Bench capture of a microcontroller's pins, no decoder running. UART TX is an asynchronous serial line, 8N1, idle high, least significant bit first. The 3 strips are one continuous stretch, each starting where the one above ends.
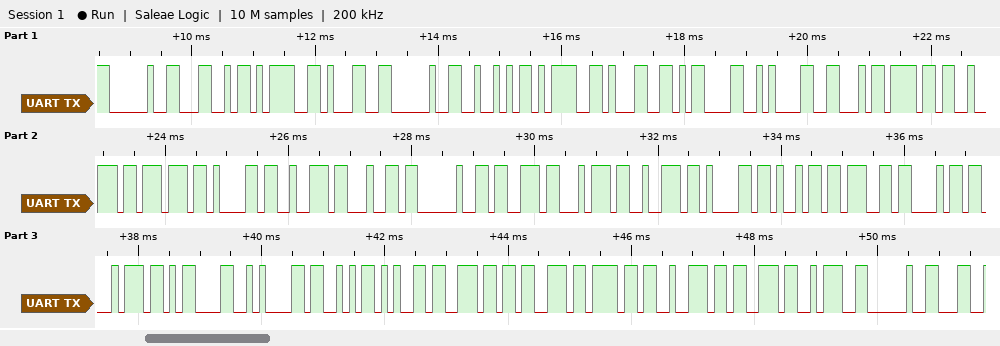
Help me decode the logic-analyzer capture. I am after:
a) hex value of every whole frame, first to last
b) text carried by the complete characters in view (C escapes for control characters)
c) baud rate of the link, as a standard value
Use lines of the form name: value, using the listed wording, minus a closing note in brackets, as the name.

hex value of every whole frame, first to last: 20 4C 3D 31 20 52 3D 31 0D 0A 46 6F 72 77 61 72 64 20 73 74 72 61 69 67 68 74 0D 0A 53 65 6E 73 6F 72 73 3A 20
text carried by the complete characters in view: " L=1 R=1\r\nForward straight\r\nSensors: "
baud rate of the link, as a standard value: 9600 baud
